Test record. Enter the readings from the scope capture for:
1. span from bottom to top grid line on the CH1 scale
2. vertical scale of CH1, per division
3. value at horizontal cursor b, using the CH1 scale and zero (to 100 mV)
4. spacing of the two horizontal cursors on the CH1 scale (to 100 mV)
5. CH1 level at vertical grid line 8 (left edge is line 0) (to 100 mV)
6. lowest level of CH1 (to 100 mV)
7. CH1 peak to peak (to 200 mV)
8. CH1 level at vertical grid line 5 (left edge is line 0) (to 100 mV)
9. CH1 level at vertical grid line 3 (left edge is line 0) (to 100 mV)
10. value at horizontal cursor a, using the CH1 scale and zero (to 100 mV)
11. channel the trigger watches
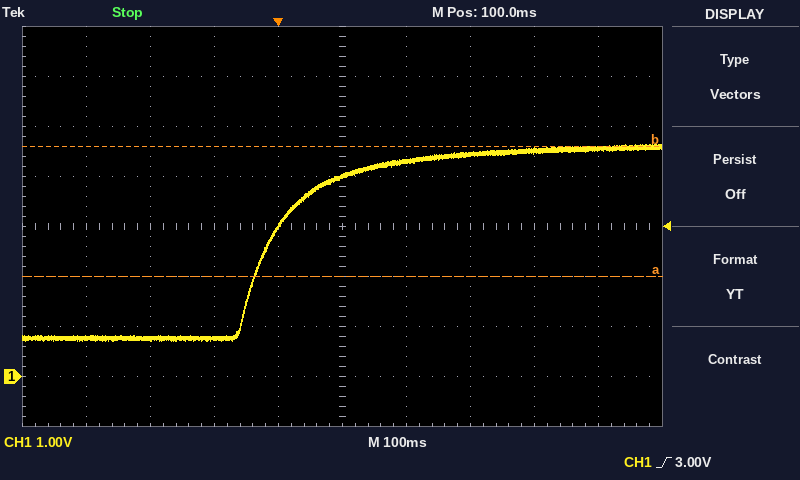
8 V
1 V
4.6 V
2.6 V
4.5 V
700 mV
4.0 V
4.0 V
800 mV
2.0 V
CH1
